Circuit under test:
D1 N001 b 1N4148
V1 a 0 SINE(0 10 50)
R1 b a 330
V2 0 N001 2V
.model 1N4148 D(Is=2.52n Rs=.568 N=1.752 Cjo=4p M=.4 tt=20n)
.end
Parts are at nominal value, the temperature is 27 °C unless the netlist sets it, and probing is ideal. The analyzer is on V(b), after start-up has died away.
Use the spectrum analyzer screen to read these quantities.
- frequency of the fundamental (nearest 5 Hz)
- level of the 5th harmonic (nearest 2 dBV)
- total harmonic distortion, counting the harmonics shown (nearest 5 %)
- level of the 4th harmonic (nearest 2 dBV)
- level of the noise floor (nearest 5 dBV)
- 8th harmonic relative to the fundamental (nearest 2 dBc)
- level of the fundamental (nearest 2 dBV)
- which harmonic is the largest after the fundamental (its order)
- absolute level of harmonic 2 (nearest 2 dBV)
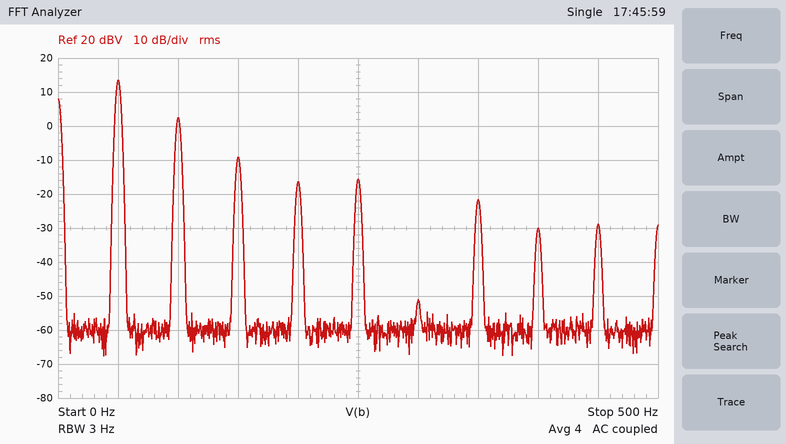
50 Hz
-16 dBV
30 %
-16 dBV
-60 dBV
-44 dBc
14 dBV
2
2 dBV
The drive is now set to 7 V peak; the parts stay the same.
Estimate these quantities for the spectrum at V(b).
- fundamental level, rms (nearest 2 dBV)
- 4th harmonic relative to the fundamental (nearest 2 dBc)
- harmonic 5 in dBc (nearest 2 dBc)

12 dBV
-44 dBc
-30 dBc
